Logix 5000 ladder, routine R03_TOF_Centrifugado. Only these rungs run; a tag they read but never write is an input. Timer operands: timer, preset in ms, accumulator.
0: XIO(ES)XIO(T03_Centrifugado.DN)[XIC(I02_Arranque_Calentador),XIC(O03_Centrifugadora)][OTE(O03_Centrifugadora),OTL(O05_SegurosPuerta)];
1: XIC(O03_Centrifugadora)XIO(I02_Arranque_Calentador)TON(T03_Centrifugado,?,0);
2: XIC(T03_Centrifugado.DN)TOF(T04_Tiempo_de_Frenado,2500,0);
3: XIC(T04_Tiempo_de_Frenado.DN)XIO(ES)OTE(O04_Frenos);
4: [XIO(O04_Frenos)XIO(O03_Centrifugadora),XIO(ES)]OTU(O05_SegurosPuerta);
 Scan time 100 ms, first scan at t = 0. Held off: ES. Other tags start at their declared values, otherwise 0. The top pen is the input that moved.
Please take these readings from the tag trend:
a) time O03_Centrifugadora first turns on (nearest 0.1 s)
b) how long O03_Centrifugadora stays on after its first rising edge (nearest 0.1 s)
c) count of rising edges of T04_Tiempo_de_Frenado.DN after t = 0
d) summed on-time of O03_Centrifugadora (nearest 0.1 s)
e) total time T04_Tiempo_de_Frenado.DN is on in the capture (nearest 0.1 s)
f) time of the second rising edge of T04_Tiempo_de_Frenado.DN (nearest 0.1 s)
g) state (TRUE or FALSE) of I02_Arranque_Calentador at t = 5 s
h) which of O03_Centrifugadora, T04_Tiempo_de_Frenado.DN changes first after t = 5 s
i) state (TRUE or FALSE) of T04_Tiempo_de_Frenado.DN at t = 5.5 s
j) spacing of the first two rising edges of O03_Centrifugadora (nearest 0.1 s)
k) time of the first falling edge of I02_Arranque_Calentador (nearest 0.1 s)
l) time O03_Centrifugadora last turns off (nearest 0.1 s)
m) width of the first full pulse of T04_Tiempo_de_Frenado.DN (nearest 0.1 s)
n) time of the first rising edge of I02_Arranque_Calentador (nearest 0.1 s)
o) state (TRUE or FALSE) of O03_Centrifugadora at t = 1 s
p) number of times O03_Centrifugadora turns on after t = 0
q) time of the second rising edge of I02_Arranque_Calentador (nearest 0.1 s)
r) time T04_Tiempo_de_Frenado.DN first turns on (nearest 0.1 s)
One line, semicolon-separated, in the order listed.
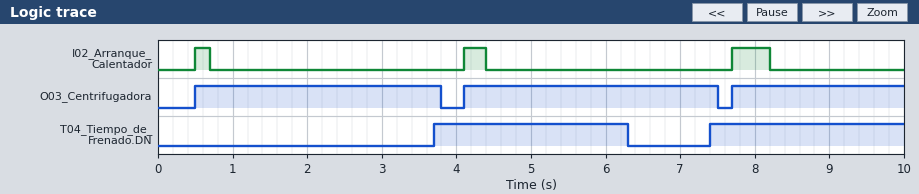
0.5 s; 3.3 s; 2; 9.0 s; 5.2 s; 7.4 s; FALSE; T04_Tiempo_de_Frenado.DN; TRUE; 3.6 s; 0.7 s; 7.5 s; 2.6 s; 0.5 s; TRUE; 3; 4.1 s; 3.7 s
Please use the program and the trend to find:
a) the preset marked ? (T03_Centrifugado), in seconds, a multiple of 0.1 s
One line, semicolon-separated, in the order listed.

3.0 s
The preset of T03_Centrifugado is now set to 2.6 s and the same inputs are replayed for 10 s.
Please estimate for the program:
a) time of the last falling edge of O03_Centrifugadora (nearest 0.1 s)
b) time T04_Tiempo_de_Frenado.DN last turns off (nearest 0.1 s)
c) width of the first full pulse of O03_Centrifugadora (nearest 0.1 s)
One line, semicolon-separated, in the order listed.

7.1 s; 9.6 s; 2.9 s
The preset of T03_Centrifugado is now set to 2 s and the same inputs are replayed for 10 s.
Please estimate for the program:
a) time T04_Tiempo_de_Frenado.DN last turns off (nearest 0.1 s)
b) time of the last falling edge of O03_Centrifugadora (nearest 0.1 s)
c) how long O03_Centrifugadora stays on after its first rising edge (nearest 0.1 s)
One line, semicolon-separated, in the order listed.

9.0 s; 6.5 s; 2.3 s
